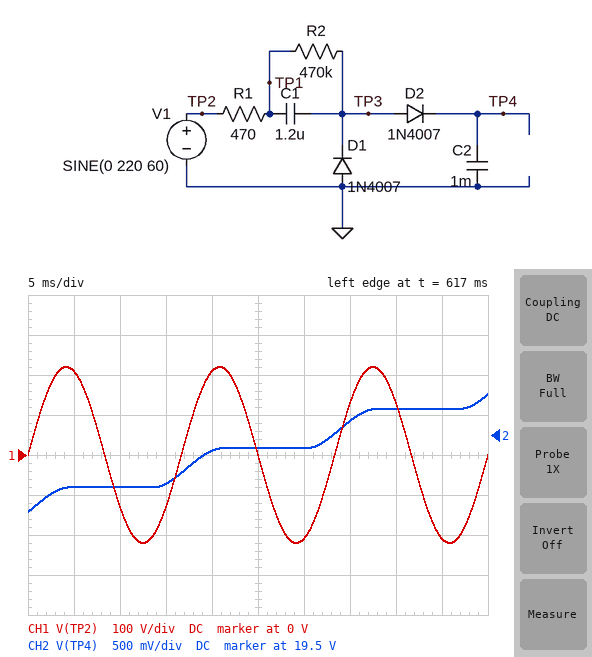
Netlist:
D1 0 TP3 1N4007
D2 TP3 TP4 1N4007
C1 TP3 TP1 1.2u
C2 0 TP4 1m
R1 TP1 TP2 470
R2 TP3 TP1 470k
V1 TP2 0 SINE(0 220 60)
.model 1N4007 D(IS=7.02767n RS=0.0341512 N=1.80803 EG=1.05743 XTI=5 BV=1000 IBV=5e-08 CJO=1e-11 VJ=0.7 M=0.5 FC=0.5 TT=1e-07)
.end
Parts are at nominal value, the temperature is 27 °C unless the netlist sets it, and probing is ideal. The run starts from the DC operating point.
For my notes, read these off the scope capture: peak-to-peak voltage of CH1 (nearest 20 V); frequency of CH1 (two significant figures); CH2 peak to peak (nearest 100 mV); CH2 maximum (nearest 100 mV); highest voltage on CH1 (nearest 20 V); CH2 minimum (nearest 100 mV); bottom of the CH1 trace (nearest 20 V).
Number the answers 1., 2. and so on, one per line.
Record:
1. 440 V
2. 60 Hz
3. 1.5 V
4. 20.0 V
5. 220 V
6. 18.5 V
7. -220 V
